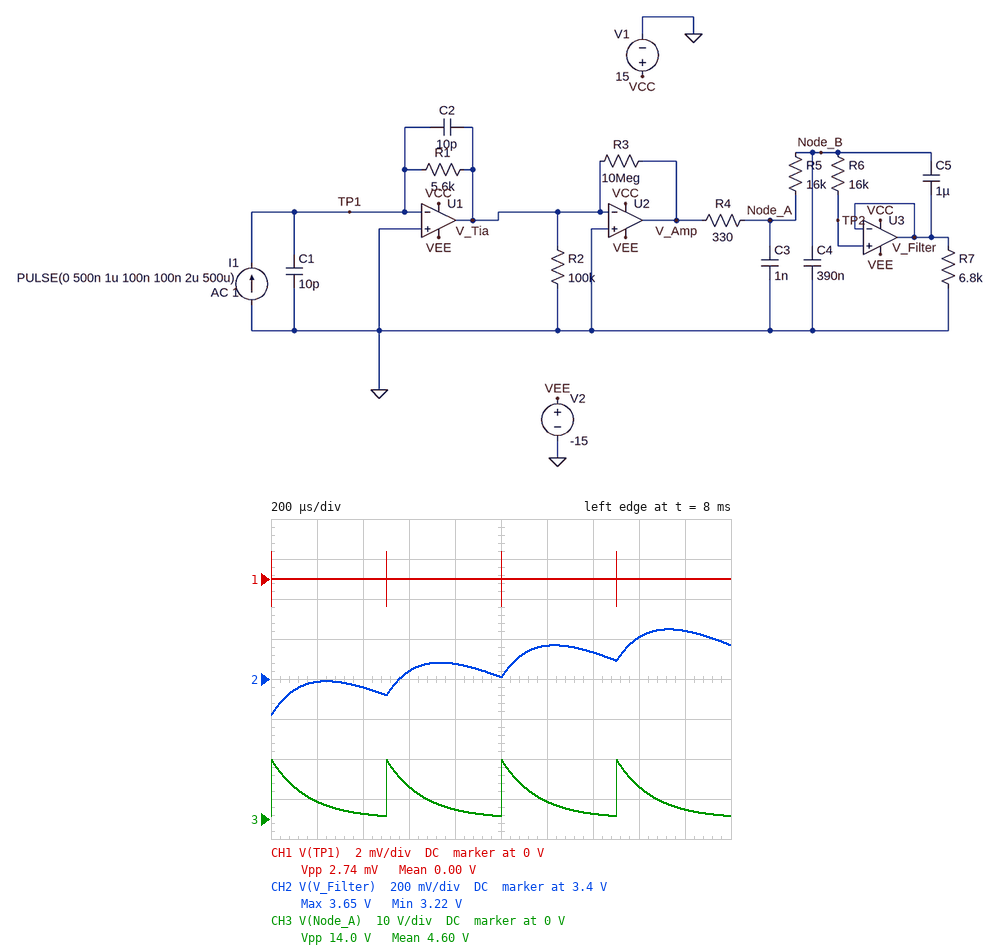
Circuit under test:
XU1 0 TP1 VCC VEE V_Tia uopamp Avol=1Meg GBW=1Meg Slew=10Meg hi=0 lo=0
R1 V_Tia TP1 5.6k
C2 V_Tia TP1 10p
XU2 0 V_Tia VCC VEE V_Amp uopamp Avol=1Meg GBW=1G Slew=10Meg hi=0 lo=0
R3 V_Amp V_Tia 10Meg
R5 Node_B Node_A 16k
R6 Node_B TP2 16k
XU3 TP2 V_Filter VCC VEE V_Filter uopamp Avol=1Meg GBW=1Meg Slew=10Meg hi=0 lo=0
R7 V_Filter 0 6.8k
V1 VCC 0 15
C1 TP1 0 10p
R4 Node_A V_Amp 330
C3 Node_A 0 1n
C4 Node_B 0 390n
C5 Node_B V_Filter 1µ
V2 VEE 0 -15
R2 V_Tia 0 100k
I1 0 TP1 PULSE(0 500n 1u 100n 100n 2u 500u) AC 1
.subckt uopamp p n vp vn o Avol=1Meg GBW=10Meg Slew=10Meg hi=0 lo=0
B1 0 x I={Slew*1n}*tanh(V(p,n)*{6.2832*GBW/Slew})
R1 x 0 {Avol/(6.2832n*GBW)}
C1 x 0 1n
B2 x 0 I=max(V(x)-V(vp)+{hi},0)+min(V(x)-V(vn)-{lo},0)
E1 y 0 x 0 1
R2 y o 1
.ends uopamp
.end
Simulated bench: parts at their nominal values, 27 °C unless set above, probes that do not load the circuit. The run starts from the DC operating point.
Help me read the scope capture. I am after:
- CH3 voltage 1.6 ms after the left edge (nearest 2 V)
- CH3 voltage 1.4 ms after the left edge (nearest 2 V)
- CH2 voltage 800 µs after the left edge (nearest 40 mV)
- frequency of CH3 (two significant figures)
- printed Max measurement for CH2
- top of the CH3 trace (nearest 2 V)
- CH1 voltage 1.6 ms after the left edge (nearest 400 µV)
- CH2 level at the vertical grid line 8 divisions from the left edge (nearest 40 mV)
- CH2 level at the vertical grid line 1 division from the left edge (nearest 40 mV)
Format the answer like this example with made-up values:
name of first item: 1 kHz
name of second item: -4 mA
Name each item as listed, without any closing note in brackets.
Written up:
CH3 voltage 1.6 ms after the left edge: 8 V
CH3 voltage 1.4 ms after the left edge: 2 V
CH2 voltage 800 µs after the left edge: 3.48 V
frequency of CH3: 2.0 kHz
printed Max measurement for CH2: 3.65 V
top of the CH3 trace: 14 V
CH1 voltage 1.6 ms after the left edge: 0 V
CH2 level at the vertical grid line 8 divisions from the left edge: 3.60 V
CH2 level at the vertical grid line 1 division from the left edge: 3.40 V
